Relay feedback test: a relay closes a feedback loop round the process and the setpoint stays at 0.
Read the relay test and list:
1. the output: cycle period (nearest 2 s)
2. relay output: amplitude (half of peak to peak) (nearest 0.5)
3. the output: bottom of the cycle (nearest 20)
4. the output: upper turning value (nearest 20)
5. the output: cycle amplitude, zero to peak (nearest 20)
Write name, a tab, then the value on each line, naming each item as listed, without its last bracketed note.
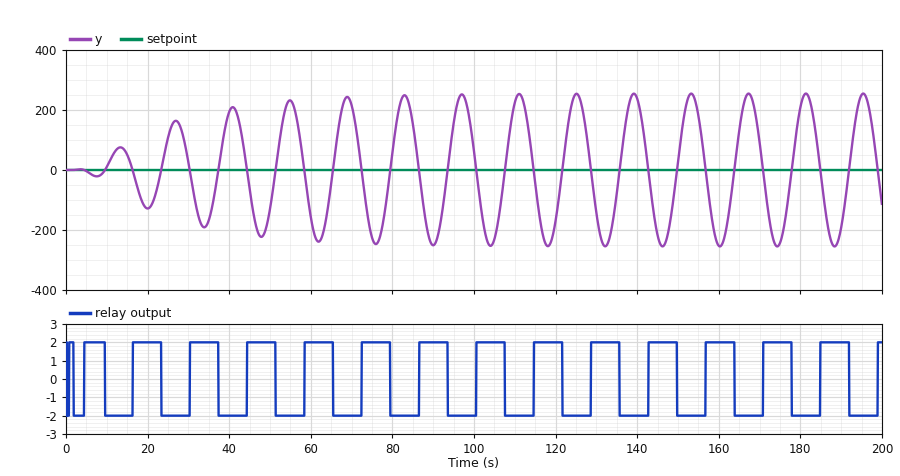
the output: cycle period	14 s
relay output: amplitude (half of peak to peak)	2.0
the output: bottom of the cycle	-260
the output: upper turning value	260
the output: cycle amplitude, zero to peak	260
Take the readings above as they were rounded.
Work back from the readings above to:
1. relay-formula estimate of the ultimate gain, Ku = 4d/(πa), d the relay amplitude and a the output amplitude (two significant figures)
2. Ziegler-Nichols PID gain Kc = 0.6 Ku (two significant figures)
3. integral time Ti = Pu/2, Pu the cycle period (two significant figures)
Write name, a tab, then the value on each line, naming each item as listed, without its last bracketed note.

relay-formula estimate of the ultimate gain, Ku = 4d/(πa), d the relay amplitude and a the output amplitude	0.0098
Ziegler-Nichols PID gain Kc = 0.6 Ku	0.0059
integral time Ti = Pu/2, Pu the cycle period	7.0 s
